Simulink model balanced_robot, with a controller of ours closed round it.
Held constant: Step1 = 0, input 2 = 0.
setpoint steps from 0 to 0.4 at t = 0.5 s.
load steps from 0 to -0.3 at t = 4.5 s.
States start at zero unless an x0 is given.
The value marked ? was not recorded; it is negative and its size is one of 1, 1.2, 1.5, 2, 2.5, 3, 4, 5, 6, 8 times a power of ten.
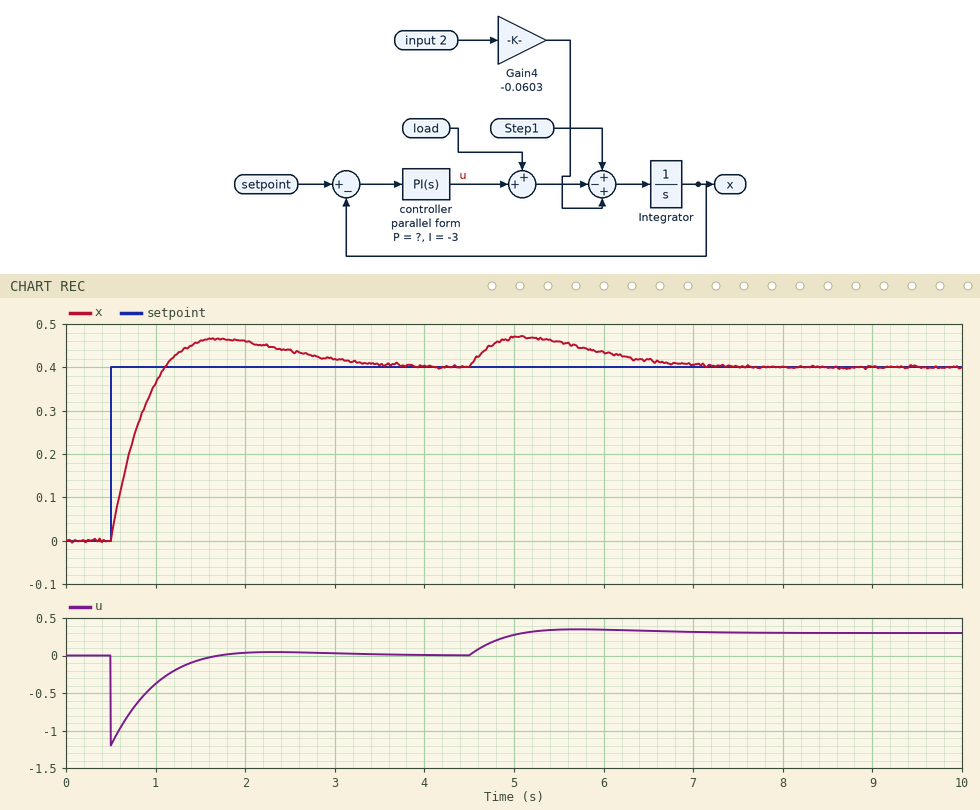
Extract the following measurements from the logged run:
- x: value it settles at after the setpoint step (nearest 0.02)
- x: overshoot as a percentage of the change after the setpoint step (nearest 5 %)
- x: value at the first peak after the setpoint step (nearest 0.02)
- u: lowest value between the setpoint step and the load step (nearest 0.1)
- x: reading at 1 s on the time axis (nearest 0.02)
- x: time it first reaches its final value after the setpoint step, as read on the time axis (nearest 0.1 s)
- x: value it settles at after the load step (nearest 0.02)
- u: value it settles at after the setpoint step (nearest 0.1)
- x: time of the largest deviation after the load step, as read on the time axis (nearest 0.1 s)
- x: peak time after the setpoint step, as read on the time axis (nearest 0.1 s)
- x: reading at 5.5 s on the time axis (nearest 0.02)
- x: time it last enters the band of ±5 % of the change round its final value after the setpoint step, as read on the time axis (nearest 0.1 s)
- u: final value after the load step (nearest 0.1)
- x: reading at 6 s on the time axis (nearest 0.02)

0.40
15 %
0.46
-1.2
0.36
1.1 s
0.40
0.0
5.1 s
1.7 s
0.46
3.0 s
0.3
0.44
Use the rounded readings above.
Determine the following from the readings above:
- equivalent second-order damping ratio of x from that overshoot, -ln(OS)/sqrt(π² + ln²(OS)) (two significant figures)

0.52
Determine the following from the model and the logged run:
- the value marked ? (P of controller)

-3
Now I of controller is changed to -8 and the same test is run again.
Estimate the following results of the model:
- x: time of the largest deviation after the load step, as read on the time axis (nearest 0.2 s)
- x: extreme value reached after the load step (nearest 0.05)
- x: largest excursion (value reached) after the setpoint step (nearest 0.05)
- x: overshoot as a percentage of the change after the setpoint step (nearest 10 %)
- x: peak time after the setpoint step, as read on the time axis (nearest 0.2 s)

5.0 s
0.45
0.50
30 %
1.4 s
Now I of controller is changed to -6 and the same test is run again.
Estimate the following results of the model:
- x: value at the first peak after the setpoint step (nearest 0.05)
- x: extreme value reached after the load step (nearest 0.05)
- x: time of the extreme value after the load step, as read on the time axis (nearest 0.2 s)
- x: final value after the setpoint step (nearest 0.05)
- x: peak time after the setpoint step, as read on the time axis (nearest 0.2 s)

0.50
0.45
5.0 s
0.40
1.4 s
